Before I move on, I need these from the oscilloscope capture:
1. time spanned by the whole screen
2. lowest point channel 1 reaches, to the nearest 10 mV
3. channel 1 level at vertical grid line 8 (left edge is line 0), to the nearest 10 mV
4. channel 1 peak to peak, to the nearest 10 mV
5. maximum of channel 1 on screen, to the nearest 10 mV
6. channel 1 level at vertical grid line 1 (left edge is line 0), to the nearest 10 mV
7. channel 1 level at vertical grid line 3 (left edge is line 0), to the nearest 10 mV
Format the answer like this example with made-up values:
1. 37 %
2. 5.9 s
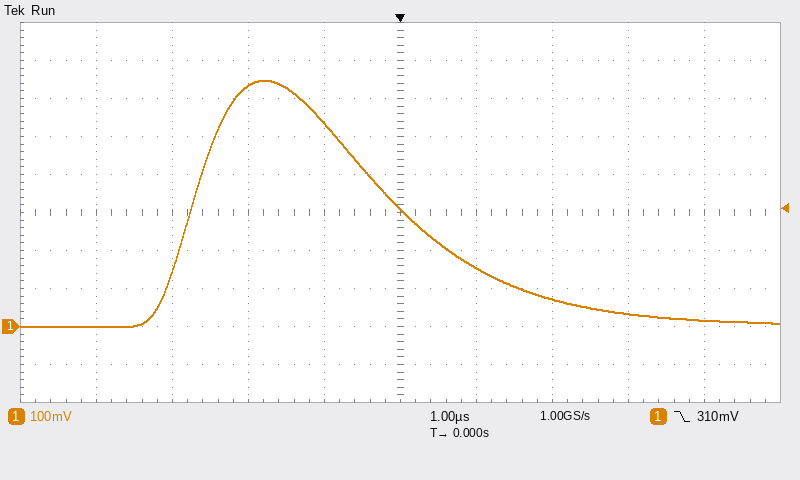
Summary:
1. 10 µs
2. 0 mV
3. 30 mV
4. 650 mV
5. 650 mV
6. 0 mV
7. 630 mV
